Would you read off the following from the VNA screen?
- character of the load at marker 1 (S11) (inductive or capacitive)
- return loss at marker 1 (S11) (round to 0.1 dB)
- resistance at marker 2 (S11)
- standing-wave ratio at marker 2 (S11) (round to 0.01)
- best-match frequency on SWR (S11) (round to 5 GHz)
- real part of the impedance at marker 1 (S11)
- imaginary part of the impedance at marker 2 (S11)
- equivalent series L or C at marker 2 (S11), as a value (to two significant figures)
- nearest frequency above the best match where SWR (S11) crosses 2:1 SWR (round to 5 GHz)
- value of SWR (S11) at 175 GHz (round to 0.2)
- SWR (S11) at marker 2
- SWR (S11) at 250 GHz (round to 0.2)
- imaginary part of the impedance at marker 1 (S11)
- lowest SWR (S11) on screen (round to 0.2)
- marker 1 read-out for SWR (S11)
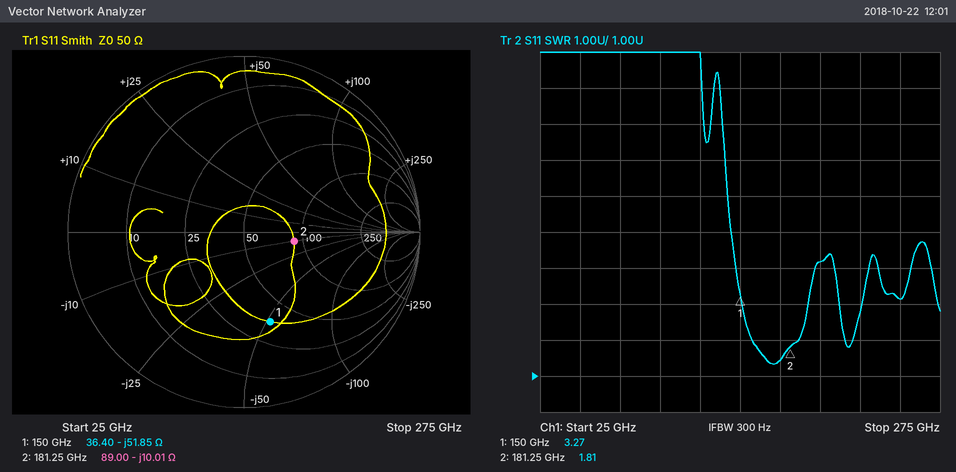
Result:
capacitive
5.5 dB
89.00 Ω
1.81
170 GHz
36.40 Ω
-10.01 Ω
88 fF
185 GHz
1.4
1.81
3.2
-51.85 Ω
1.4
3.27
